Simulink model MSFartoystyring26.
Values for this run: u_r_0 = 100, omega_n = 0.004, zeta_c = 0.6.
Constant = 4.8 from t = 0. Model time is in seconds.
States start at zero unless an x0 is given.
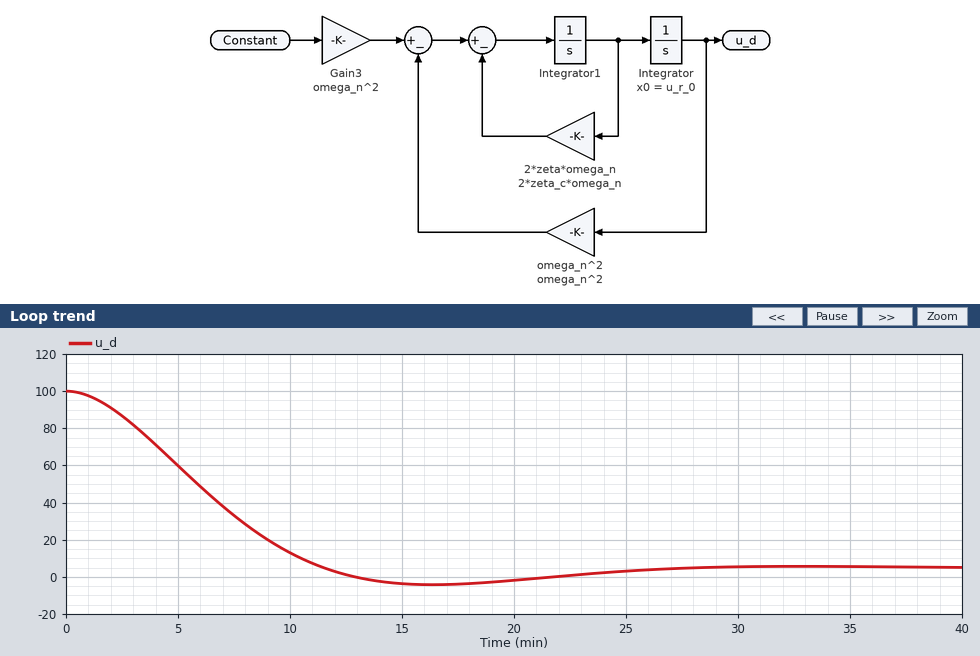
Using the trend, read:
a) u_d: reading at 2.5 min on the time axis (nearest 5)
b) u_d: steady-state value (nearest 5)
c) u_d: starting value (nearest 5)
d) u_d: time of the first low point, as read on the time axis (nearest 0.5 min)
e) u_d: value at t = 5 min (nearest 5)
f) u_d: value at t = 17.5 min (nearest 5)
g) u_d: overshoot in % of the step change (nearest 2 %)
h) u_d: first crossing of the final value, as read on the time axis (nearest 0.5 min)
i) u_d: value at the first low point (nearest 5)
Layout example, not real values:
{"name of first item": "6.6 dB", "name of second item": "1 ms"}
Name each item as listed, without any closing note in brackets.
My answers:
{"u_d: reading at 2.5 min on the time axis": "85", "u_d: steady-state value": "5", "u_d: starting value": "100", "u_d: time of the first low point, as read on the time axis": "16.5 min", "u_d: value at t = 5 min": "60", "u_d: value at t = 17.5 min": "-5", "u_d: overshoot in % of the step change": "10 %", "u_d: first crossing of the final value, as read on the time axis": "11.5 min", "u_d: value at the first low point": "-5"}
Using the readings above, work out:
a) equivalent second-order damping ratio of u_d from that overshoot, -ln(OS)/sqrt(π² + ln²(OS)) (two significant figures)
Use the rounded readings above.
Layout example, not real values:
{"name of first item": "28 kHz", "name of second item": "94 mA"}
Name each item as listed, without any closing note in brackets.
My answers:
{"equivalent second-order damping ratio of u_d from that overshoot, -ln(OS)/sqrt(π² + ln²(OS))": "0.59"}
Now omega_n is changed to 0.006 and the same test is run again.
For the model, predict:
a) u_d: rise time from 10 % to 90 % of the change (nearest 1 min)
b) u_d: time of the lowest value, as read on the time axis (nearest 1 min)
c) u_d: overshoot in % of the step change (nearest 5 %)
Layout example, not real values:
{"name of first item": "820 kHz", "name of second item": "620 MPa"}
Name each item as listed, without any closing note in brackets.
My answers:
{"u_d: rise time from 10 % to 90 % of the change": "5 min", "u_d: time of the lowest value, as read on the time axis": "11 min", "u_d: overshoot in % of the step change": "10 %"}
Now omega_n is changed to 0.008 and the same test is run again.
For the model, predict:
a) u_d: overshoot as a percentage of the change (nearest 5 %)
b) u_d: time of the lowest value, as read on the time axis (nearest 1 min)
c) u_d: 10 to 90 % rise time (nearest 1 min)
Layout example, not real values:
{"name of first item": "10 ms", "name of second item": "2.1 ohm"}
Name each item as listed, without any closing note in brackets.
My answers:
{"u_d: overshoot as a percentage of the change": "10 %", "u_d: time of the lowest value, as read on the time axis": "8 min", "u_d: 10 to 90 % rise time": "4 min"}
